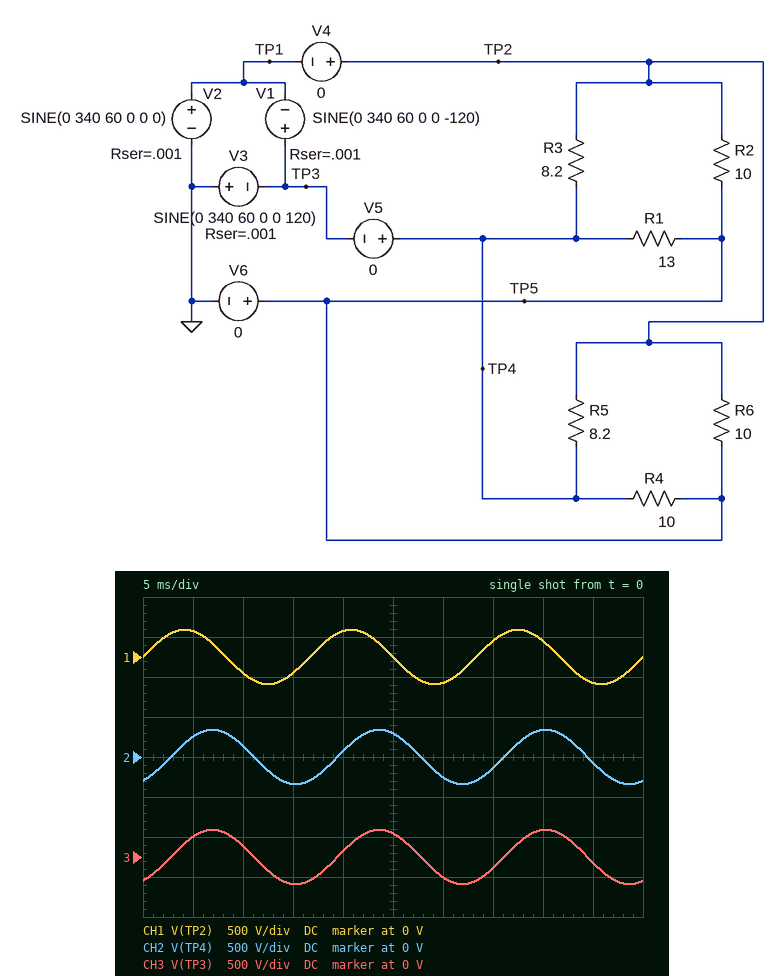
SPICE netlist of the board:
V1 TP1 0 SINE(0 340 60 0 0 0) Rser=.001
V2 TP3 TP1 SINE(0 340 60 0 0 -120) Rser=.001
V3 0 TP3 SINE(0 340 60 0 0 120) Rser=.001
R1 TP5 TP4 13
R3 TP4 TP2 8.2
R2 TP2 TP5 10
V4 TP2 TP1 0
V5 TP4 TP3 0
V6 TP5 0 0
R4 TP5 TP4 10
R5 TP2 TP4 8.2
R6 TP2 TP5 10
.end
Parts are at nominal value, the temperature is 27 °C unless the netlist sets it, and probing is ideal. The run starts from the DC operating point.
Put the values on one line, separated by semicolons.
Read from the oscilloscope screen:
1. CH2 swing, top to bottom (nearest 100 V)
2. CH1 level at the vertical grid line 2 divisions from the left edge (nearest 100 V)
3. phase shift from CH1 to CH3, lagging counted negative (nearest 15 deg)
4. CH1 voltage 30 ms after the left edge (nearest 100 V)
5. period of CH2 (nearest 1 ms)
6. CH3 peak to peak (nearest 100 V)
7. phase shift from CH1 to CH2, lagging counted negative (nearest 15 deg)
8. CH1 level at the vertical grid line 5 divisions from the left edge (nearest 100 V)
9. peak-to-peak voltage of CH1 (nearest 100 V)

700 V; -200 V; -60 deg; -300 V; 17 ms; 700 V; -60 deg; 0 V; 700 V
